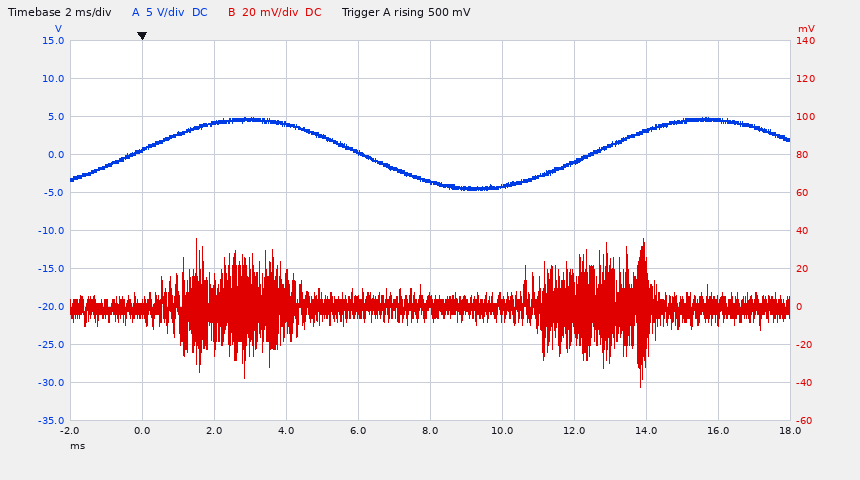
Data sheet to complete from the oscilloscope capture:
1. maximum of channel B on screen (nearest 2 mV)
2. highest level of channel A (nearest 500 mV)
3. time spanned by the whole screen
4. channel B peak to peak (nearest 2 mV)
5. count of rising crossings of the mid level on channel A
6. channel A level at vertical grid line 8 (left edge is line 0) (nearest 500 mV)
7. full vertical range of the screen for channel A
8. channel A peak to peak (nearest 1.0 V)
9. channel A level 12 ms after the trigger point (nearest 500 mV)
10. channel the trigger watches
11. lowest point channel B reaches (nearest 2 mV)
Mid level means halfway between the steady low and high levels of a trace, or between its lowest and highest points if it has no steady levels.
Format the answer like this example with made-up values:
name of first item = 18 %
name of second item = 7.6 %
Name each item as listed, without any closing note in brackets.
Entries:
maximum of channel B on screen = 36 mV
highest level of channel A = 5.0 V
time spanned by the whole screen = 20 ms
channel B peak to peak = 78 mV
count of rising crossings of the mid level on channel A = 2
channel A level at vertical grid line 8 (left edge is line 0) = 3.0 V
full vertical range of the screen for channel A = 50 V
channel A peak to peak = 10.0 V
channel A level 12 ms after the trigger point = -1.0 V
channel the trigger watches = channel A
lowest point channel B reaches = -42 mV
